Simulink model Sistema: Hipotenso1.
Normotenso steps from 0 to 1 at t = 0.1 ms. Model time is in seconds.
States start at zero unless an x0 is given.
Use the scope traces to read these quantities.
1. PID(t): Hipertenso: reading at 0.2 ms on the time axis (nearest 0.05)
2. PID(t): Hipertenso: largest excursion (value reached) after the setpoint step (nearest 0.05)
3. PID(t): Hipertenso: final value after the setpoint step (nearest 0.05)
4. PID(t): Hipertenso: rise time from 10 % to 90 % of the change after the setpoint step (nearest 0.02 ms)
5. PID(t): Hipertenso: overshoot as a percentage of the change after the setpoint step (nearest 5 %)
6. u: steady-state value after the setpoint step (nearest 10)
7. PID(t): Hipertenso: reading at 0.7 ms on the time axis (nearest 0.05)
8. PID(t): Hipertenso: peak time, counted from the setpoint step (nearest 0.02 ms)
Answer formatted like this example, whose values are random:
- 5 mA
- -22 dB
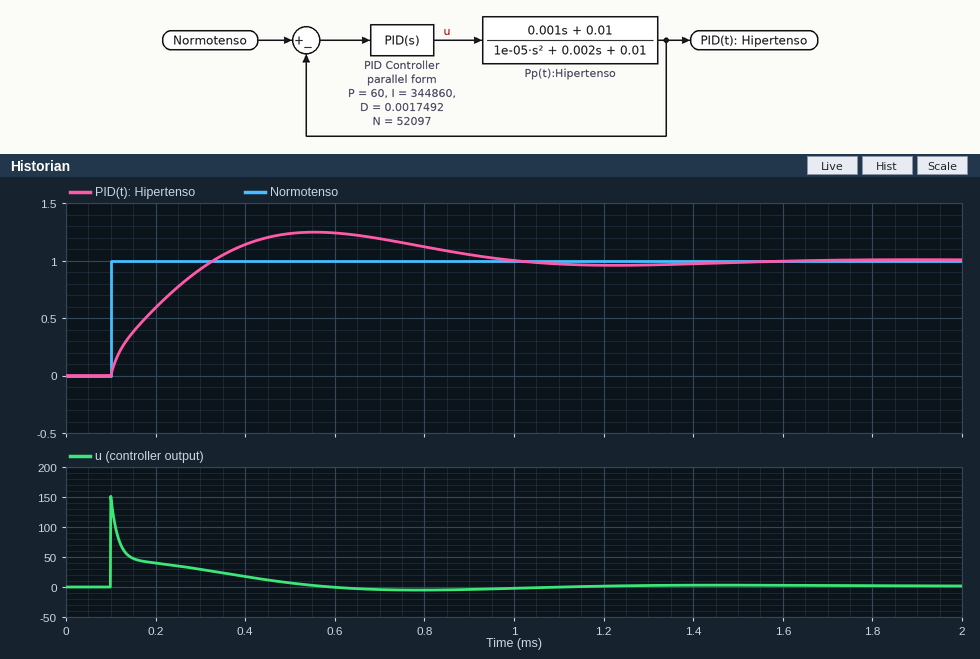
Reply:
- 0.60
- 1.25
- 1.00
- 0.18 ms
- 25 %
- 0
- 1.20
- 0.46 ms
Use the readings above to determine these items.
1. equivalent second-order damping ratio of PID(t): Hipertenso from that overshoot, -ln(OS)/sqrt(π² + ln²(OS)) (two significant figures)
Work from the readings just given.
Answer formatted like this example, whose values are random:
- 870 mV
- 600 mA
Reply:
- 0.40
